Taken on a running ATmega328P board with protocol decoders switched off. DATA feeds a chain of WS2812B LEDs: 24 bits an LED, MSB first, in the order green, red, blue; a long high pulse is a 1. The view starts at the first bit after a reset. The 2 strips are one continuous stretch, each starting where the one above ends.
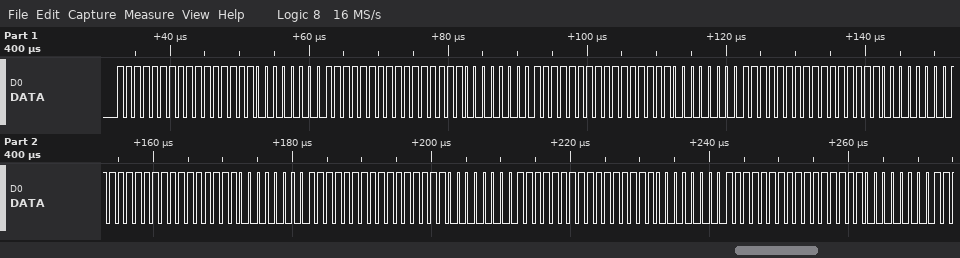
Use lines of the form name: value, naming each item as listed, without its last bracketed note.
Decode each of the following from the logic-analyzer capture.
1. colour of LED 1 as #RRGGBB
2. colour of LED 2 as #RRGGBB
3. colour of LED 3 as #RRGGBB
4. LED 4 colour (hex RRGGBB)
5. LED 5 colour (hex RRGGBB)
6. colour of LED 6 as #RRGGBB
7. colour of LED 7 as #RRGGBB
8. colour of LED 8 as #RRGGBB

colour of LED 1 as #RRGGBB: #FFFF00
colour of LED 2 as #RRGGBB: #FFFF00
colour of LED 3 as #RRGGBB: #FFFF00
LED 4 colour: #FFFF00
LED 5 colour: #FFFF00
colour of LED 6 as #RRGGBB: #FFFF00
colour of LED 7 as #RRGGBB: #FFFF00
colour of LED 8 as #RRGGBB: #FFFF00
